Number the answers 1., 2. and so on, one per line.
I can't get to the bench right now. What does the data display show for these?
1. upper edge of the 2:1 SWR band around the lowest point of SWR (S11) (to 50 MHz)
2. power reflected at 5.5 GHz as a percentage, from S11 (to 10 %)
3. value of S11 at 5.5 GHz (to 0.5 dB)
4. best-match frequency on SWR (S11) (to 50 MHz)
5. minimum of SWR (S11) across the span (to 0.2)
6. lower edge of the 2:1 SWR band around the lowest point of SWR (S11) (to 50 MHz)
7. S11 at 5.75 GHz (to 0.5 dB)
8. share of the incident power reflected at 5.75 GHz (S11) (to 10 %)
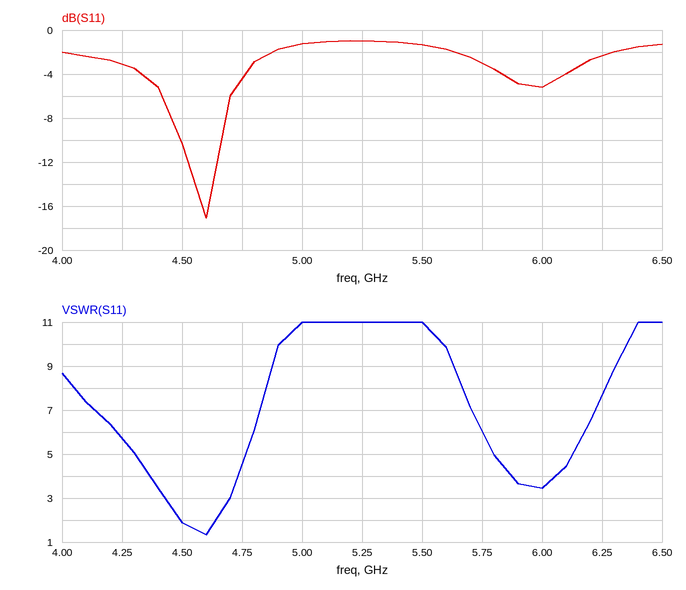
1. 4.65 GHz
2. 70 %
3. -1.5 dB
4. 4.60 GHz
5. 1.4
6. 4.50 GHz
7. -3.0 dB
8. 50 %
